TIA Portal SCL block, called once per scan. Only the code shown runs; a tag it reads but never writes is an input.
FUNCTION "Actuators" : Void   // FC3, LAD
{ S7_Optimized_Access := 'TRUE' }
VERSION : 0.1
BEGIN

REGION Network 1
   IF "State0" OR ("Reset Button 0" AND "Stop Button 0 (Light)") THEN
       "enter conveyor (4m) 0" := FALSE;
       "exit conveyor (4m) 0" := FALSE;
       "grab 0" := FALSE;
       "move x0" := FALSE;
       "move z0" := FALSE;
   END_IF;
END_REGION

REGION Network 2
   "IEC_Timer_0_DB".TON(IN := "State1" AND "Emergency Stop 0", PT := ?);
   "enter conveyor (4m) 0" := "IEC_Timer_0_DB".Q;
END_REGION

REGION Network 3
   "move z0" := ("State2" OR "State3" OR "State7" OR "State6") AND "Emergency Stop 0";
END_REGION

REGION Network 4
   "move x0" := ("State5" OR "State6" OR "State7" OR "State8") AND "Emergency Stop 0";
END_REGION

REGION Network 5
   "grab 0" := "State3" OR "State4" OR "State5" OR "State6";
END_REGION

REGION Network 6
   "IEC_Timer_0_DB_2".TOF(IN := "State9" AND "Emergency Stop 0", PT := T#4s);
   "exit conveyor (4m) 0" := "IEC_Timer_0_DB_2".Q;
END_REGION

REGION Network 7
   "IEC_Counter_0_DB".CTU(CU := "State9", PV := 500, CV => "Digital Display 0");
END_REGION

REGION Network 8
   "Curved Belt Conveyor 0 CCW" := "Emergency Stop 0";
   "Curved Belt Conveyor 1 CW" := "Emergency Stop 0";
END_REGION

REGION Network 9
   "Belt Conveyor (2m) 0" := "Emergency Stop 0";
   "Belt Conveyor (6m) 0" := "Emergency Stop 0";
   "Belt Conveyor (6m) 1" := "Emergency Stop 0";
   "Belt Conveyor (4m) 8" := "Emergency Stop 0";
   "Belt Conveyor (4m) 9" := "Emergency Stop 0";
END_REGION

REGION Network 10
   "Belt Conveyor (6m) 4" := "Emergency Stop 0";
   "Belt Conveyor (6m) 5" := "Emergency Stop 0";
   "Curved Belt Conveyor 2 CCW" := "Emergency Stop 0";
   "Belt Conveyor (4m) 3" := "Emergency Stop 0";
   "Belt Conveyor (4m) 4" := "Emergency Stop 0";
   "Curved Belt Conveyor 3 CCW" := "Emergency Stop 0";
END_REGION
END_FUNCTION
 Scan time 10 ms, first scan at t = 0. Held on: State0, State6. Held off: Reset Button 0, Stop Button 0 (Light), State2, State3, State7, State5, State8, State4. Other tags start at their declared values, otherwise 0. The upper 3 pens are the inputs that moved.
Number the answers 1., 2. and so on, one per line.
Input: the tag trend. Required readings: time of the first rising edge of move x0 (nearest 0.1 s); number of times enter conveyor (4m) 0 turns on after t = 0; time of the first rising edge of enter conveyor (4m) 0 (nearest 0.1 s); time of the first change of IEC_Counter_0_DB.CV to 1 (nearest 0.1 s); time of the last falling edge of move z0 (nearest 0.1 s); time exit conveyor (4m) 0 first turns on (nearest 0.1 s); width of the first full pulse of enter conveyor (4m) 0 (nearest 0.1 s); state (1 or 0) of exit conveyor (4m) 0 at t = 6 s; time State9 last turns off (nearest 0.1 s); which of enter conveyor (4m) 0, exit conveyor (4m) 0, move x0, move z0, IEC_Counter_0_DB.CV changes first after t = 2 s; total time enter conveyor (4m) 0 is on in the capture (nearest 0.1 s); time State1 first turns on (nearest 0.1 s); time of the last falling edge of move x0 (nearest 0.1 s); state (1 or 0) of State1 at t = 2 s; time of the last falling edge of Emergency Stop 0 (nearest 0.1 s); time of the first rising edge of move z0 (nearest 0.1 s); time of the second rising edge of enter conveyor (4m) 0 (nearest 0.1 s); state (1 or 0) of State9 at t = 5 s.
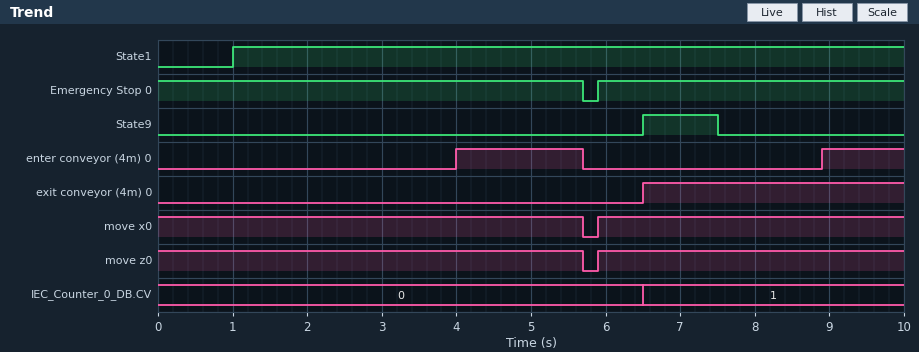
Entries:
1. 5.9 s
2. 2
3. 4.0 s
4. 6.5 s
5. 5.7 s
6. 6.5 s
7. 1.7 s
8. 0
9. 7.5 s
10. enter conveyor (4m) 0
11. 2.8 s
12. 1.0 s
13. 5.7 s
14. 1
15. 5.7 s
16. 5.9 s
17. 8.9 s
18. 0
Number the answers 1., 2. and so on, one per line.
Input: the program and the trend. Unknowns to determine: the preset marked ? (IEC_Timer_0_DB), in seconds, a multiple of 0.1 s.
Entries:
1. 3.0 s
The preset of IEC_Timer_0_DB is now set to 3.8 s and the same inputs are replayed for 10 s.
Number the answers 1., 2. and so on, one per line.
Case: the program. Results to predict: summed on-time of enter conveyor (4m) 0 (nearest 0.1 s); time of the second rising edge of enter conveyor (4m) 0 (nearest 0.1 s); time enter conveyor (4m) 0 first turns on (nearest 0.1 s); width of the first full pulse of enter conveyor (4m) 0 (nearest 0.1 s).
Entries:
1. 1.2 s
2. 9.7 s
3. 4.8 s
4. 0.9 s
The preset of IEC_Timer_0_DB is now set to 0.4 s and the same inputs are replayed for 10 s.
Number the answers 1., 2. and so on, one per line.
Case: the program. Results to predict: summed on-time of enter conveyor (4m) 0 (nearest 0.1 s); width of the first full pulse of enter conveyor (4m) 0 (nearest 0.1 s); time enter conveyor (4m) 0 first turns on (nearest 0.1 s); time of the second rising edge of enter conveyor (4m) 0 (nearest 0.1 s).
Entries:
1. 8.0 s
2. 4.3 s
3. 1.4 s
4. 6.3 s
